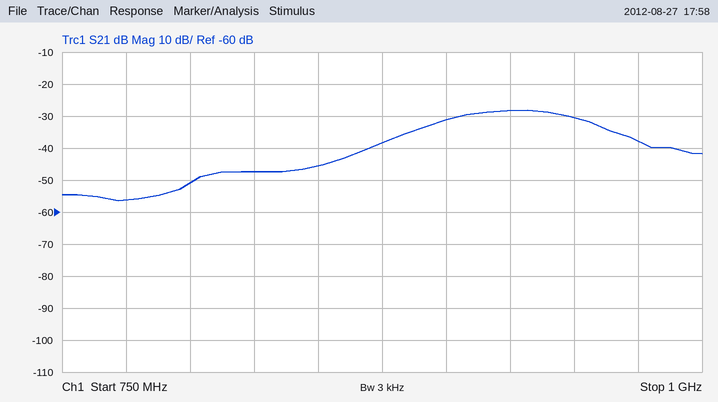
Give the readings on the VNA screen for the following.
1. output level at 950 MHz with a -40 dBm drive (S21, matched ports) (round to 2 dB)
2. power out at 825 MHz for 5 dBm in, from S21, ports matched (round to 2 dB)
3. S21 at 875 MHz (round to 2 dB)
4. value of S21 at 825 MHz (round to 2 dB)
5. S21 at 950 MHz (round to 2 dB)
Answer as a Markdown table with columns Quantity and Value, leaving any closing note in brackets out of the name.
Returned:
| Quantity | Value |
|---|---|
| output level at 950 MHz with a -40 dBm drive (S21, matched ports) | -70 dBm |
| power out at 825 MHz for 5 dBm in, from S21, ports matched | -42 dBm |
| S21 at 875 MHz | -38 dB |
| value of S21 at 825 MHz | -48 dB |
| S21 at 950 MHz | -30 dB |
